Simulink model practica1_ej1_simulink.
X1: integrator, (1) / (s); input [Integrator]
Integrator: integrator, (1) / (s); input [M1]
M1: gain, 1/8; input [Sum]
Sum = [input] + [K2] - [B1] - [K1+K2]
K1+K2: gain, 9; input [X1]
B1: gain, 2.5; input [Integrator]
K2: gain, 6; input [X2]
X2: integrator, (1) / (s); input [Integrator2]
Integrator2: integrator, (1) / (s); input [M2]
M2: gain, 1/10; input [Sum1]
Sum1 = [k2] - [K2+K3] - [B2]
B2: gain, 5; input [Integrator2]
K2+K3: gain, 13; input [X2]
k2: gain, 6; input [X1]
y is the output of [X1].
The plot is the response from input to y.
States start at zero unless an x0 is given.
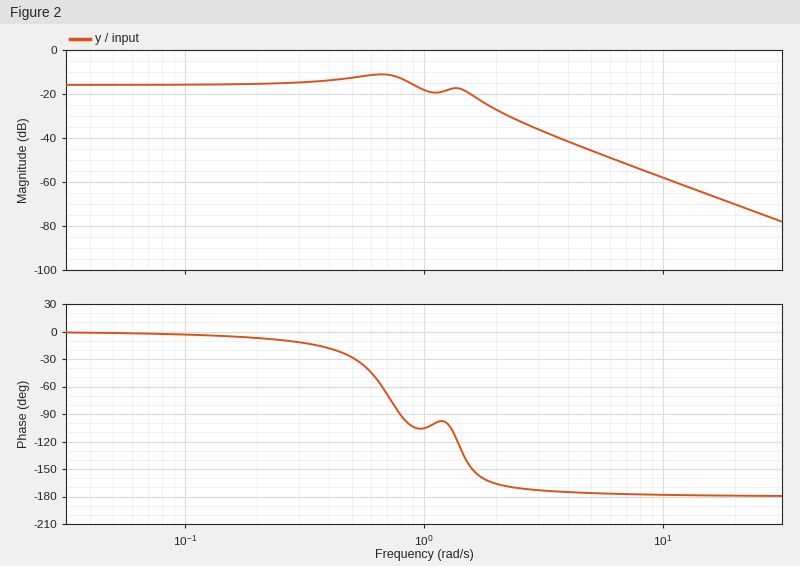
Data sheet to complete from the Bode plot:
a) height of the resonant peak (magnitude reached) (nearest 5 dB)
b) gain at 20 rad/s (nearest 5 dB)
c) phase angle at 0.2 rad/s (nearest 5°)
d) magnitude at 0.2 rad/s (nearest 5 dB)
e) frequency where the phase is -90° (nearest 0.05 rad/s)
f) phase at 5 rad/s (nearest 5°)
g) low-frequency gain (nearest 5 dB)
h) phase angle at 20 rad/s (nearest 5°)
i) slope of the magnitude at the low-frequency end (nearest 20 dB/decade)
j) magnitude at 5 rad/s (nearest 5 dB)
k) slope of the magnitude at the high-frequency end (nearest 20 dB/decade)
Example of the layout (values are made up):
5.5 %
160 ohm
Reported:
-10 dB
-70 dB
-5°
-15 dB
0.80 rad/s
-175°
-15 dB
-180°
0 dB/decade
-45 dB
-40 dB/decade
